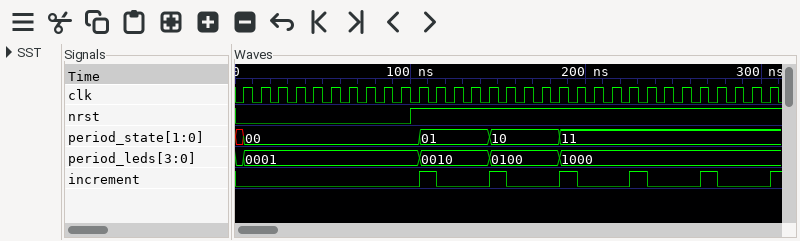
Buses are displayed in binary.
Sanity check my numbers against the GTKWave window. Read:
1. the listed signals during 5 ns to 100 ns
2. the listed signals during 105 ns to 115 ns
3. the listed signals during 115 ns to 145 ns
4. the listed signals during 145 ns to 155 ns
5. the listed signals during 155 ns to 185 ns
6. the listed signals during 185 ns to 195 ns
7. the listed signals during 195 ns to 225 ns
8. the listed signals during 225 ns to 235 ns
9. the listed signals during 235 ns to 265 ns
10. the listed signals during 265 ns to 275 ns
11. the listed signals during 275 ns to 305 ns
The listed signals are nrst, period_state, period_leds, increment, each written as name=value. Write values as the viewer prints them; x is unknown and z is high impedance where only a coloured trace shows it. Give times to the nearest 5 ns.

nrst=0, period_state=00, period_leds=0001, increment=0
nrst=1, period_state=01, period_leds=0010, increment=1
nrst=1, period_state=01, period_leds=0010, increment=0
nrst=1, period_state=10, period_leds=0100, increment=1
nrst=1, period_state=10, period_leds=0100, increment=0
nrst=1, period_state=11, period_leds=1000, increment=1
nrst=1, period_state=11, period_leds=1000, increment=0
nrst=1, period_state=11, period_leds=1000, increment=1
nrst=1, period_state=11, period_leds=1000, increment=0
nrst=1, period_state=11, period_leds=1000, increment=1
nrst=1, period_state=11, period_leds=1000, increment=0
